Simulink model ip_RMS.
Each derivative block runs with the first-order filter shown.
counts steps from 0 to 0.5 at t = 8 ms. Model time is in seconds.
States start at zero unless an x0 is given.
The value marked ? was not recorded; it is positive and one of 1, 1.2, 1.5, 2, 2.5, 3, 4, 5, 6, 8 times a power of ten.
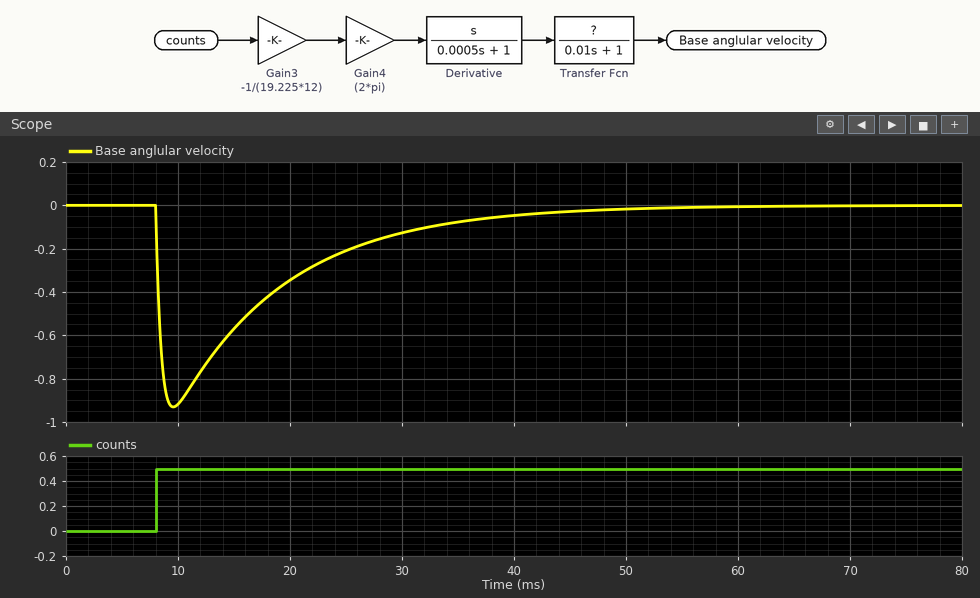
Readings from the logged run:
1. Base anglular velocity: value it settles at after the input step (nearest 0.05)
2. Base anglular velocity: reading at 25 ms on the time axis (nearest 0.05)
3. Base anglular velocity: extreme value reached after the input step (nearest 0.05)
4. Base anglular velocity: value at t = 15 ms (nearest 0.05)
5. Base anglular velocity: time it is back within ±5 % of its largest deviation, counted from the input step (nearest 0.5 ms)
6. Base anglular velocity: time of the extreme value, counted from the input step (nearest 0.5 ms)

0.00
-0.20
-0.95
-0.55
32.0 ms
1.5 ms
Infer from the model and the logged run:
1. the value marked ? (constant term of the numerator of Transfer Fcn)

0.8
